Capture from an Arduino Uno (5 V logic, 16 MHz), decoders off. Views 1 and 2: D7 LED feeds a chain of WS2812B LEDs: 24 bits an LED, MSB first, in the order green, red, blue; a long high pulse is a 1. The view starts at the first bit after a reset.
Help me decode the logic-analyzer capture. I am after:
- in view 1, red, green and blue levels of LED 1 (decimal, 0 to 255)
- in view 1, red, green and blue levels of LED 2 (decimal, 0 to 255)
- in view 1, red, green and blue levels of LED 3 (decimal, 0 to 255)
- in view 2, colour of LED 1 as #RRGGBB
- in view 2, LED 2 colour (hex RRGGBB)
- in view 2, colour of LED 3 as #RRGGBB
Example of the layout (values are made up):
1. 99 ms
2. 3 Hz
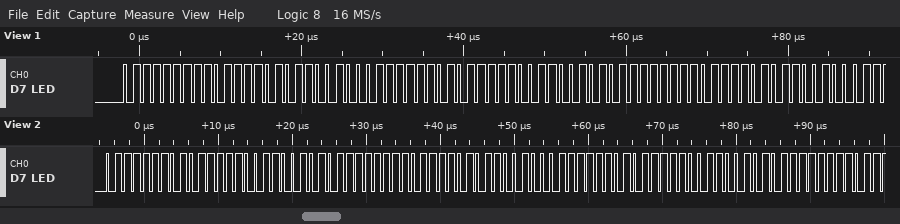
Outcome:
1. 189, 127, 100
2. 190, 126, 101
3. 189, 127, 100
4. #BE7E65
5. #BD7F64
6. #BE7E65
